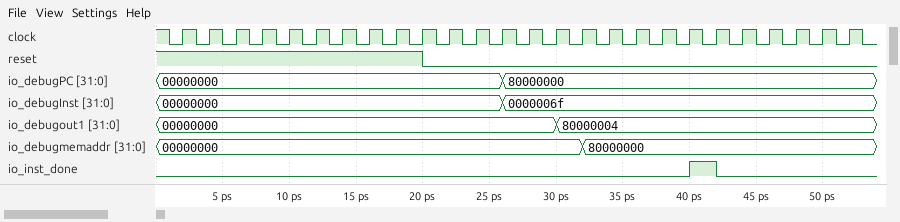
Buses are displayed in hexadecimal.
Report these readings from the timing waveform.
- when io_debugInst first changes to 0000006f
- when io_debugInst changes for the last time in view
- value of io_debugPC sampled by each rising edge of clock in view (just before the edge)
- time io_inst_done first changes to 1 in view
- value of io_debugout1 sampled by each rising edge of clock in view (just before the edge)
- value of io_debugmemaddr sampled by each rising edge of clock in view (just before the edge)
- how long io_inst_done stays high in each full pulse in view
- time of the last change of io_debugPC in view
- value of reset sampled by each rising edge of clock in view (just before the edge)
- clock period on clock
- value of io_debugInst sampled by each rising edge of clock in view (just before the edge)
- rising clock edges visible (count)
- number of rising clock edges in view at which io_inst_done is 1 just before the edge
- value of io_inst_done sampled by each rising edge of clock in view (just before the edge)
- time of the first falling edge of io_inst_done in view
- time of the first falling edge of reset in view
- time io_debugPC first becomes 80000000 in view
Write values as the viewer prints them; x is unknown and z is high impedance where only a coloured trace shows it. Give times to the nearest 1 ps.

26 ps
26 ps
00000000, 00000000, 00000000, 00000000, 00000000, 00000000, 00000000, 00000000, 00000000, 00000000, 00000000, 00000000, 00000000, 80000000, 80000000, 80000000, 80000000, 80000000, 80000000, 80000000, 80000000, 80000000, 80000000, 80000000, 80000000, 80000000
40 ps
00000000, 00000000, 00000000, 00000000, 00000000, 00000000, 00000000, 00000000, 00000000, 00000000, 00000000, 00000000, 00000000, 00000000, 00000000, 80000004, 80000004, 80000004, 80000004, 80000004, 80000004, 80000004, 80000004, 80000004, 80000004, 80000004
00000000, 00000000, 00000000, 00000000, 00000000, 00000000, 00000000, 00000000, 00000000, 00000000, 00000000, 00000000, 00000000, 00000000, 00000000, 00000000, 80000000, 80000000, 80000000, 80000000, 80000000, 80000000, 80000000, 80000000, 80000000, 80000000
2 ps
26 ps
1 1 1 1 1 1 1 1 1 1 0 0 0 0 0 0 0 0 0 0 0 0 0 0 0 0
2 ps
00000000, 00000000, 00000000, 00000000, 00000000, 00000000, 00000000, 00000000, 00000000, 00000000, 00000000, 00000000, 00000000, 0000006f, 0000006f, 0000006f, 0000006f, 0000006f, 0000006f, 0000006f, 0000006f, 0000006f, 0000006f, 0000006f, 0000006f, 0000006f
26
1
0 0 0 0 0 0 0 0 0 0 0 0 0 0 0 0 0 0 0 0 1 0 0 0 0 0
42 ps
20 ps
26 ps
